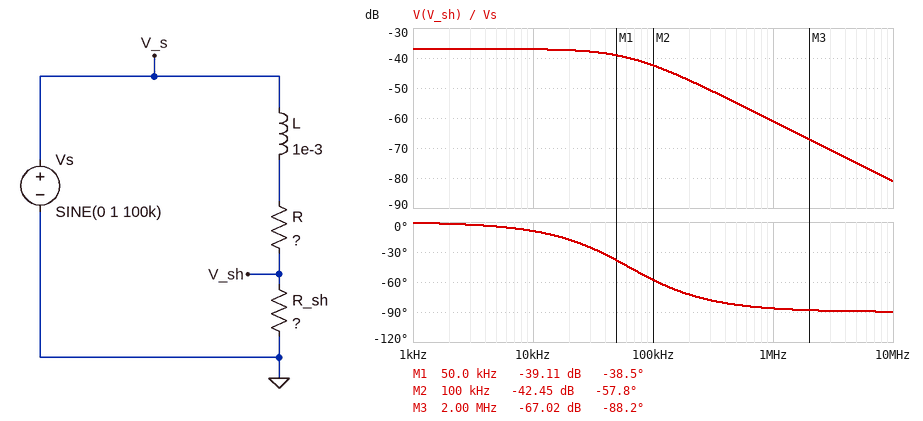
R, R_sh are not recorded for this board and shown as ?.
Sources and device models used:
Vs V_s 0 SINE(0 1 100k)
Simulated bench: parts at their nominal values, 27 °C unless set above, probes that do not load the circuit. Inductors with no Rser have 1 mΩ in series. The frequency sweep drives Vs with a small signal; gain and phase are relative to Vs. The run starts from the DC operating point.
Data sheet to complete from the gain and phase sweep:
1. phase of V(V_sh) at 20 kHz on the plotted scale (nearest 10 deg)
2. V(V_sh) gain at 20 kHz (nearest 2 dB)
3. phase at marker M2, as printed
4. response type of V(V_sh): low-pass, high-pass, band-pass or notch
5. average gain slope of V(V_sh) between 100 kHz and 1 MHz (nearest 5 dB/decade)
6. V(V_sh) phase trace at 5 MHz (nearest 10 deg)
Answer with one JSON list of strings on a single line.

["-20 deg", "-38 dB", "-57.8 deg", "low-pass", "-20 dB/decade", "-90 deg"]
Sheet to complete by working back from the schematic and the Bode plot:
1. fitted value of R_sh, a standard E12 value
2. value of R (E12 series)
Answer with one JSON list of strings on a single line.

["5.6 Ω", "390 Ω"]
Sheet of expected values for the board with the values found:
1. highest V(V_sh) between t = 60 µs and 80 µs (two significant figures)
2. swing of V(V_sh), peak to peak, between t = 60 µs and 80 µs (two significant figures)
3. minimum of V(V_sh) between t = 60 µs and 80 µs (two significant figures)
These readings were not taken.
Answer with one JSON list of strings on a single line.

["7.5 mV", "15 mV", "-7.5 mV"]
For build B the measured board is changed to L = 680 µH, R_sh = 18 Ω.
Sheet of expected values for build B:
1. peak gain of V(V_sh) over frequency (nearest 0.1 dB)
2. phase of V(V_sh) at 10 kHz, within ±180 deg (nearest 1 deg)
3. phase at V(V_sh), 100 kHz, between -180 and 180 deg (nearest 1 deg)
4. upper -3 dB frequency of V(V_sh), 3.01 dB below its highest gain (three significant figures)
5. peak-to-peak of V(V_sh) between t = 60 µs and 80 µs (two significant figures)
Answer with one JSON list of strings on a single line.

["-27.1 dB", "-6 deg", "-46 deg", "95.5 kHz", "61 mV"]
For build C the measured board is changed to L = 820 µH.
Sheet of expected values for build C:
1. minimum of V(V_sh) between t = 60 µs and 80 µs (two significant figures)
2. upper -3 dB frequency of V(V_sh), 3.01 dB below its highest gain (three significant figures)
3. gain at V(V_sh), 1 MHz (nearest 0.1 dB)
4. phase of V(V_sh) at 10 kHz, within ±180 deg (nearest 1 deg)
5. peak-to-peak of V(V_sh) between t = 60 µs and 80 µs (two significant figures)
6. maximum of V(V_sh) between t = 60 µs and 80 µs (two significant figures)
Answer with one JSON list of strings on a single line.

["-8.6 mV", "76.8 kHz", "-59.3 dB", "-7 deg", "17 mV", "8.6 mV"]
